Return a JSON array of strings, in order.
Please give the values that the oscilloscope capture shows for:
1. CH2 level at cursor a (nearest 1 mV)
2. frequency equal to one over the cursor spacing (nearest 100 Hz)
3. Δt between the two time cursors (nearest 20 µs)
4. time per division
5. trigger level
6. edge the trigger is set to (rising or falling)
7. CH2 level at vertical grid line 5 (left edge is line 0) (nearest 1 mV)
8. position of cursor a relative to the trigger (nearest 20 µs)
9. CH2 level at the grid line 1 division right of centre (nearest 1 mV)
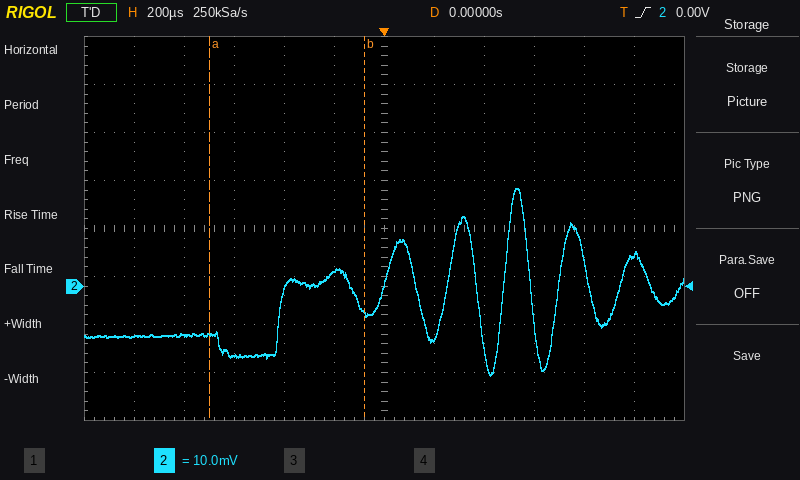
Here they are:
["-10 mV", "1.6 kHz", "620 µs", "200 µs", "0.00 V", "rising", "3 mV", "-700 µs", "-11 mV"]
